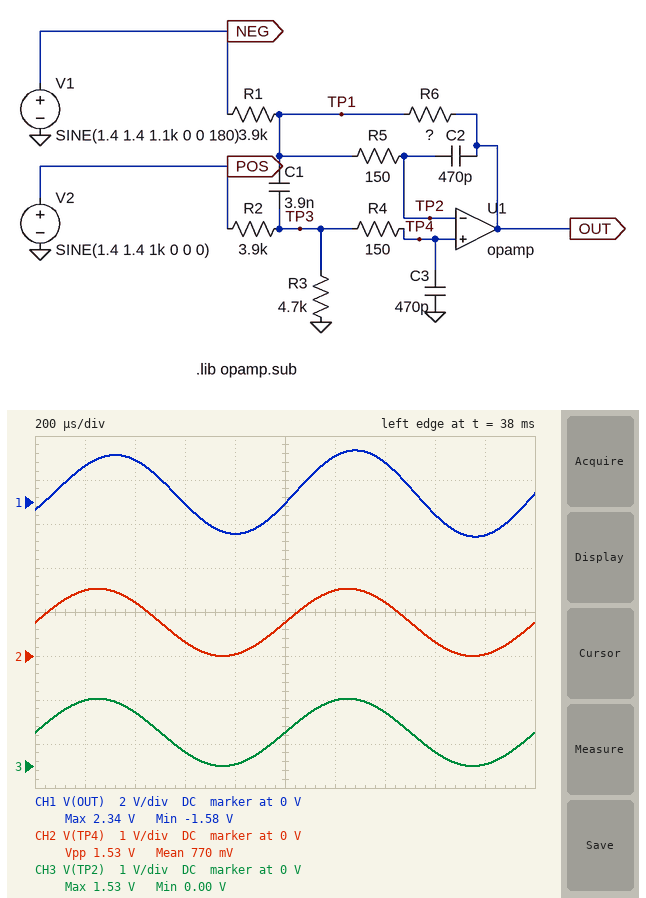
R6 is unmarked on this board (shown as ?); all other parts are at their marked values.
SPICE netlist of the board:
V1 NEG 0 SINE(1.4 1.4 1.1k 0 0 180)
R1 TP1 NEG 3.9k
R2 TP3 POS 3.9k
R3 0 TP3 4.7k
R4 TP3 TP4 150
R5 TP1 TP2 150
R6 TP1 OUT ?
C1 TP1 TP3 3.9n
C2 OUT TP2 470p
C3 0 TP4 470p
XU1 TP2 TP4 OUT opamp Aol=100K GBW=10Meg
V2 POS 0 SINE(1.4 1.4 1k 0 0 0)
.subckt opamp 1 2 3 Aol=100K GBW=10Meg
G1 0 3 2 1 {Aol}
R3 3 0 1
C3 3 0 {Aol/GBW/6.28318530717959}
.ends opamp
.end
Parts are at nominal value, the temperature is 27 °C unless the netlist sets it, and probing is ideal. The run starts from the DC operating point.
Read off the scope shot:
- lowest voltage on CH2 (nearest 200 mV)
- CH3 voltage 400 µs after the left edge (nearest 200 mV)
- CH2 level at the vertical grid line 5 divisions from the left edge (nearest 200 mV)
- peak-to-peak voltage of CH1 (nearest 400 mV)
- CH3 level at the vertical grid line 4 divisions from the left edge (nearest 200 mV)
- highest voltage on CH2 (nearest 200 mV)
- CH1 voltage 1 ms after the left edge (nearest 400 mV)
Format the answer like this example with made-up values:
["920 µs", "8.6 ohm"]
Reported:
["0 V", "1.2 V", "800 mV", "4.0 V", "0 V", "1.6 V", "0 V"]
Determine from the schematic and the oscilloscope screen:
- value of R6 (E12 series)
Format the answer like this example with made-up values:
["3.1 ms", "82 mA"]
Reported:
["2.2 kΩ"]
